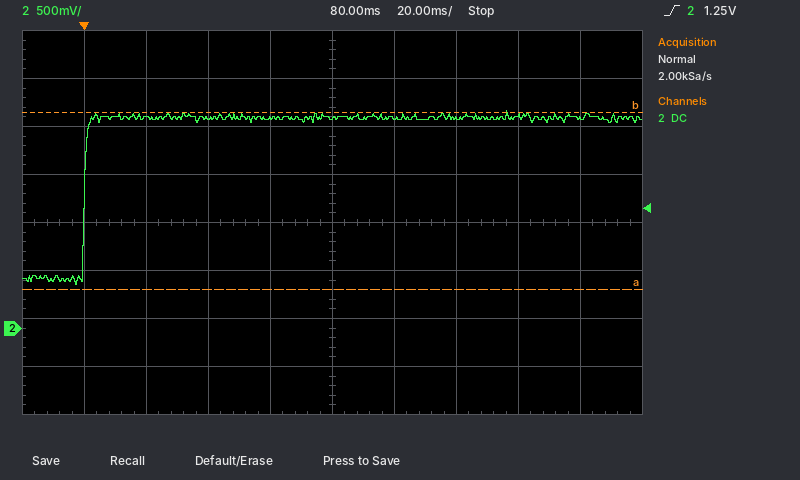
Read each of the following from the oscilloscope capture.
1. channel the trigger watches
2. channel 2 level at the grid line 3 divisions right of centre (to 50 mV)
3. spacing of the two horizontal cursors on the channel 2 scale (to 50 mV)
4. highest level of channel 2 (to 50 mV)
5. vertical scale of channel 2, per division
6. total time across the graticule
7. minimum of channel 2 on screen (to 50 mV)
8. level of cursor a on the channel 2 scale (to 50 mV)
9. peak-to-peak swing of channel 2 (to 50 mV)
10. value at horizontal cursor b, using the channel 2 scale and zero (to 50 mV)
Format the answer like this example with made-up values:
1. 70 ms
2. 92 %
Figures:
1. channel 2
2. 2.20 V
3. 1.85 V
4. 2.25 V
5. 500 mV
6. 200 ms
7. 450 mV
8. 400 mV
9. 1.80 V
10. 2.25 V
